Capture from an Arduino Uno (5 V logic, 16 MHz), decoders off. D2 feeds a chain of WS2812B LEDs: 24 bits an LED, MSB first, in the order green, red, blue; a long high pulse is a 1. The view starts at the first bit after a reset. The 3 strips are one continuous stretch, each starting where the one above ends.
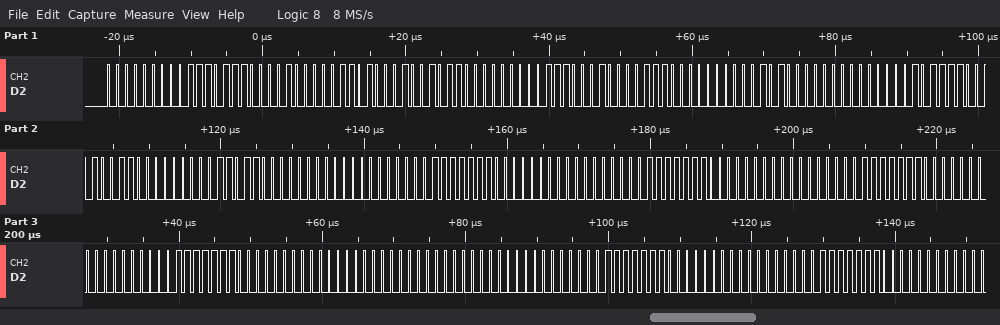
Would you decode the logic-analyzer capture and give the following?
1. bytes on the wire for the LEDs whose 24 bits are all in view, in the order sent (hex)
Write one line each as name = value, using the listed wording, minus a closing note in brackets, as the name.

bytes on the wire for the LEDs whose 24 bits are all in view, in the order sent = 00 77 08 34 4B 00 71 0E 00 50 00 2F 13 00 6C 00 00 7F 00 00 7F 00 00 7F 00 00 7F 00 00 00 00 00 7F 00 00 7F
